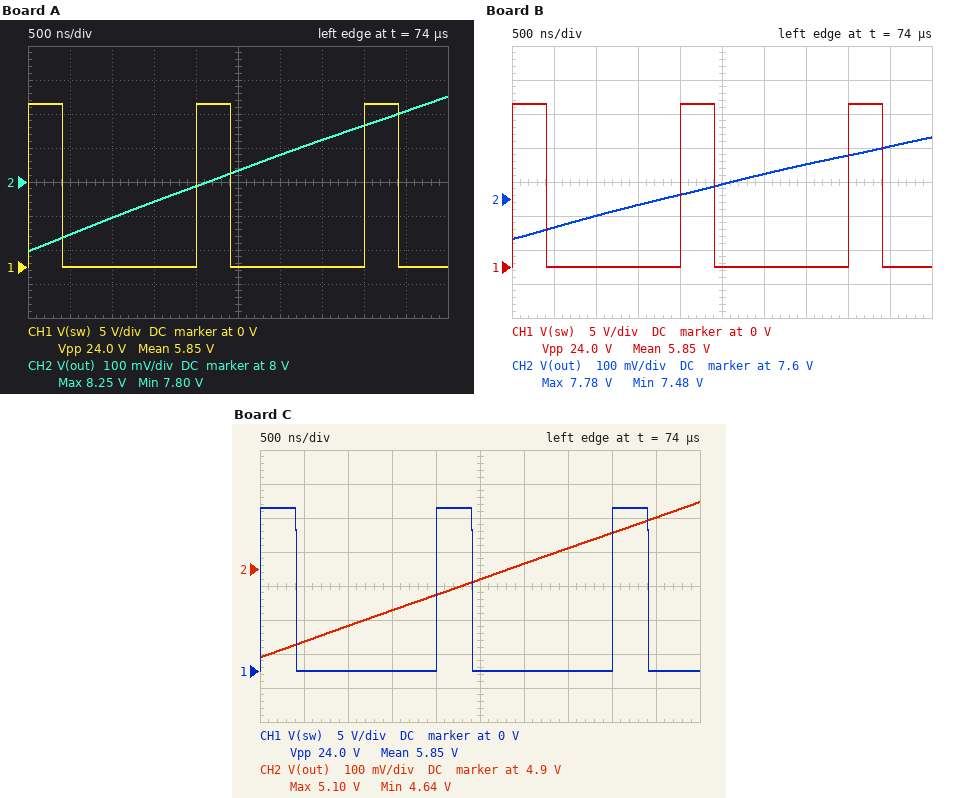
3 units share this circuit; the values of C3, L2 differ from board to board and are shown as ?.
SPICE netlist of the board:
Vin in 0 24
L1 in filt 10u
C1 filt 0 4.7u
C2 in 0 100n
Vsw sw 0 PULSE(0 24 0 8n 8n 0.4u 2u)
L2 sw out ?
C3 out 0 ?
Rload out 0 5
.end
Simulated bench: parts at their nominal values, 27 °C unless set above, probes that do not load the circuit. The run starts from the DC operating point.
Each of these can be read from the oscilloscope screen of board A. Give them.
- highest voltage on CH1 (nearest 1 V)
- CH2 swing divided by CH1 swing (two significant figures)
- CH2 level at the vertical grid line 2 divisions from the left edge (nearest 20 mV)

24 V
0.019
7.90 V
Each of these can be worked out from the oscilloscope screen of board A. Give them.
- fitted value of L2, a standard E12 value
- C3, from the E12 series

15 µH
68 µF
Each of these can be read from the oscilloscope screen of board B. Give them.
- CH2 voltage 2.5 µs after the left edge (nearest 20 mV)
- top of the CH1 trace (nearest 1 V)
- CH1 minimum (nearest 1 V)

7.64 V
24 V
0 V
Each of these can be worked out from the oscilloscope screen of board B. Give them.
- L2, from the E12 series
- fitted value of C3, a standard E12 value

39 µH
22 µF
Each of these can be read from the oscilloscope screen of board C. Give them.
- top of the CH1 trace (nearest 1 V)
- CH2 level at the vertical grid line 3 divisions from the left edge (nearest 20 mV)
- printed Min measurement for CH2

24 V
4.78 V
4.64 V
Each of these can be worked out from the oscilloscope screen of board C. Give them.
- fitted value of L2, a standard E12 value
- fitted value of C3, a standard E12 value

39 µH
56 µF
